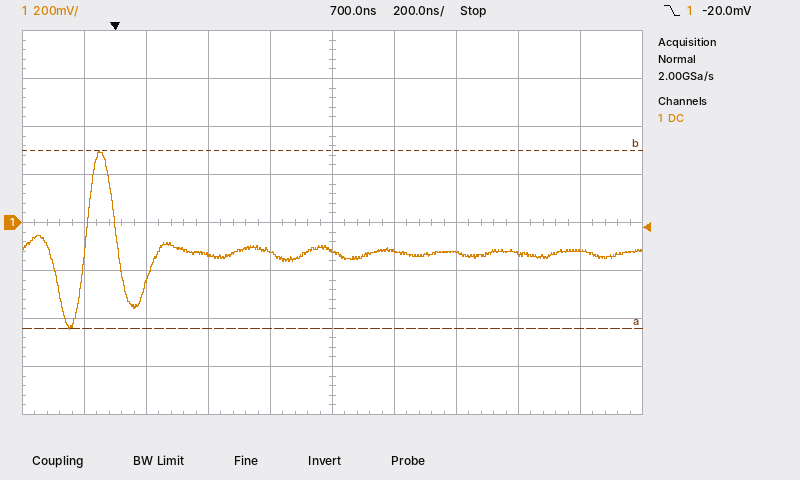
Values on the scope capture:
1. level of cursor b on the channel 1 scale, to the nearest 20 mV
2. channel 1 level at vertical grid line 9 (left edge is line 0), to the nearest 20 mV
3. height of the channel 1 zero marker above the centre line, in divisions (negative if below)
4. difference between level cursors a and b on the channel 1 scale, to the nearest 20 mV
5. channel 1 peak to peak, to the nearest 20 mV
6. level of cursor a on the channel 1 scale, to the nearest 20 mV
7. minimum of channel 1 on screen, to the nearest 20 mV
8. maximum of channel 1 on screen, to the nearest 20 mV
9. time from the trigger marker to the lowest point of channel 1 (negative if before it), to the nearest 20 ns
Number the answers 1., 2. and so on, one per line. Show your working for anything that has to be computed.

1. 300 mV
2. -120 mV
3. 0.0 div
4. 740 mV
5. 300 mV − (-440 mV) = 740 mV
6. -440 mV
7. -440 mV
8. 300 mV
9. -140 ns
